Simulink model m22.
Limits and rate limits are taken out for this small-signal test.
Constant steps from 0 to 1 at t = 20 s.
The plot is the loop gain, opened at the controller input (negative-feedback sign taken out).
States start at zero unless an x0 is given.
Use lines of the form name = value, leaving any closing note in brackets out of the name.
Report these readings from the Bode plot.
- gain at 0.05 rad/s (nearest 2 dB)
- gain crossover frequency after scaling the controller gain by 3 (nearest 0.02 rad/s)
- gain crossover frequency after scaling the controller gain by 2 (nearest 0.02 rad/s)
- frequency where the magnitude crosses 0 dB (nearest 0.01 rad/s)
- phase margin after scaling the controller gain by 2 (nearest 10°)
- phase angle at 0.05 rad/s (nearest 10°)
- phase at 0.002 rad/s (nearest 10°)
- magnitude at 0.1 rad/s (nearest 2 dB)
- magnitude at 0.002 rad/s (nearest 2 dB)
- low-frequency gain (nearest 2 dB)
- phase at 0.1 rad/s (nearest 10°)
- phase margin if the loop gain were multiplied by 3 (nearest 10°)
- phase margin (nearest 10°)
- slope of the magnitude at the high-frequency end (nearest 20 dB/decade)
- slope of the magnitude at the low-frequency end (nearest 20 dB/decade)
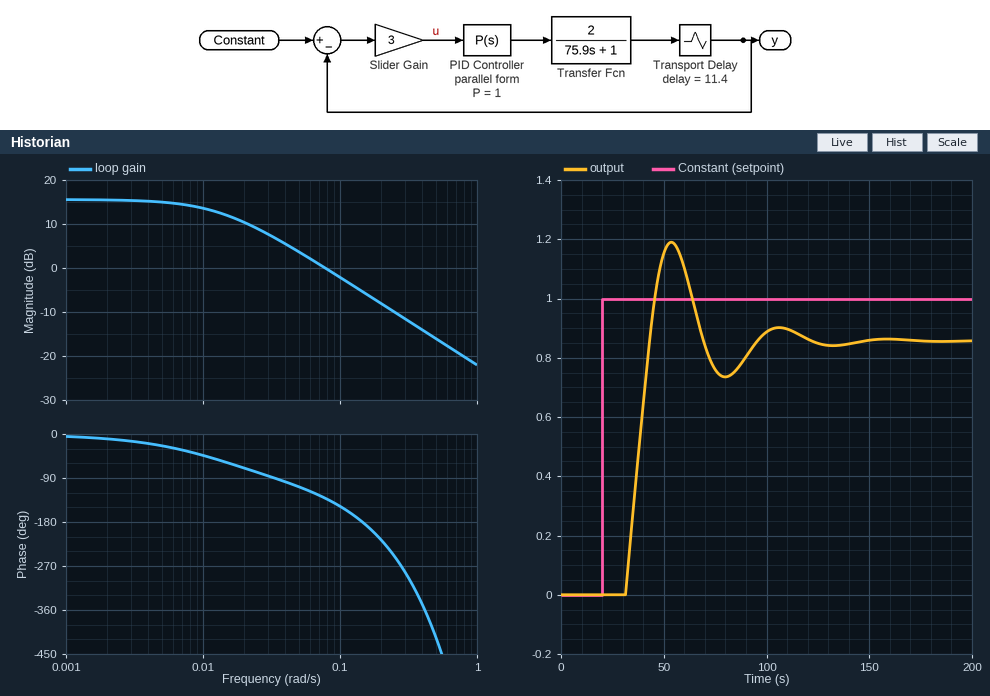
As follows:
gain at 0.05 rad/s = 4 dB
gain crossover frequency after scaling the controller gain by 3 = 0.24 rad/s
gain crossover frequency after scaling the controller gain by 2 = 0.16 rad/s
frequency where the magnitude crosses 0 dB = 0.08 rad/s
phase margin after scaling the controller gain by 2 = -10°
phase angle at 0.05 rad/s = -110°
phase at 0.002 rad/s = -10°
magnitude at 0.1 rad/s = -2 dB
magnitude at 0.002 rad/s = 16 dB
low-frequency gain = 16 dB
phase at 0.1 rad/s = -150°
phase margin if the loop gain were multiplied by 3 = -60°
phase margin = 50°
slope of the magnitude at the high-frequency end = -20 dB/decade
slope of the magnitude at the low-frequency end = 0 dB/decade
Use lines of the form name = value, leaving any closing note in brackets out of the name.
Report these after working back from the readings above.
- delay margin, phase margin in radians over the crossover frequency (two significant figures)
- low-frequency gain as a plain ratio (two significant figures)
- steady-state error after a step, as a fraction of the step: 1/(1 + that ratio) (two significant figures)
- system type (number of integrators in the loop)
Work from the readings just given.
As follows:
delay margin, phase margin in radians over the crossover frequency = 11 s
low-frequency gain as a plain ratio = 6.3
steady-state error after a step, as a fraction of the step: 1/(1 + that ratio) = 0.14
system type = 0
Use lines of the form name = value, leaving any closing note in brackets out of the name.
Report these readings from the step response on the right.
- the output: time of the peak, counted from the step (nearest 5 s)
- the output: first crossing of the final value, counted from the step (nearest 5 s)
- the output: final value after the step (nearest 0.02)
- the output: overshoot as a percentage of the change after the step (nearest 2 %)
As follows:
the output: time of the peak, counted from the step = 35 s
the output: first crossing of the final value, counted from the step = 25 s
the output: final value after the step = 0.86
the output: overshoot as a percentage of the change after the step = 38 %
